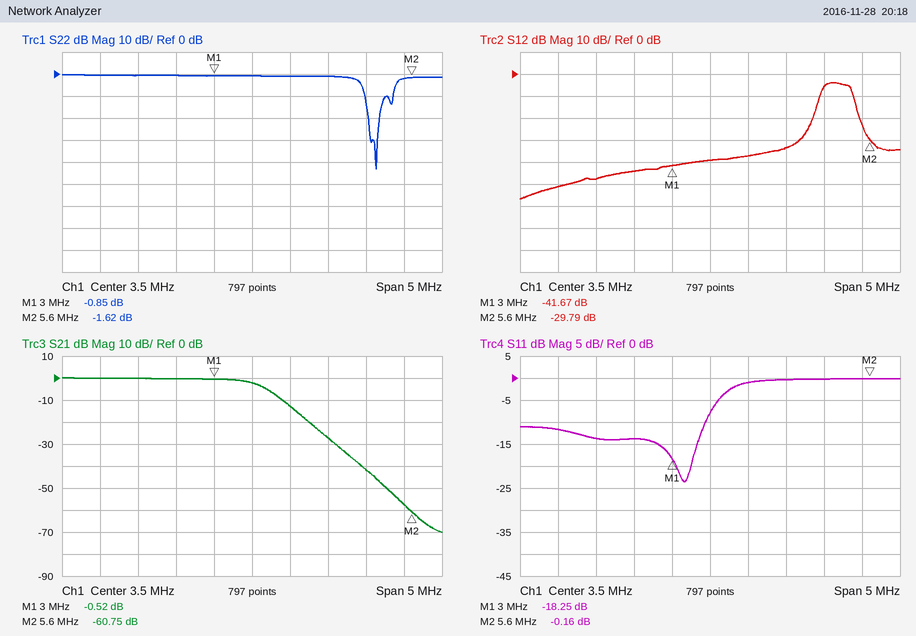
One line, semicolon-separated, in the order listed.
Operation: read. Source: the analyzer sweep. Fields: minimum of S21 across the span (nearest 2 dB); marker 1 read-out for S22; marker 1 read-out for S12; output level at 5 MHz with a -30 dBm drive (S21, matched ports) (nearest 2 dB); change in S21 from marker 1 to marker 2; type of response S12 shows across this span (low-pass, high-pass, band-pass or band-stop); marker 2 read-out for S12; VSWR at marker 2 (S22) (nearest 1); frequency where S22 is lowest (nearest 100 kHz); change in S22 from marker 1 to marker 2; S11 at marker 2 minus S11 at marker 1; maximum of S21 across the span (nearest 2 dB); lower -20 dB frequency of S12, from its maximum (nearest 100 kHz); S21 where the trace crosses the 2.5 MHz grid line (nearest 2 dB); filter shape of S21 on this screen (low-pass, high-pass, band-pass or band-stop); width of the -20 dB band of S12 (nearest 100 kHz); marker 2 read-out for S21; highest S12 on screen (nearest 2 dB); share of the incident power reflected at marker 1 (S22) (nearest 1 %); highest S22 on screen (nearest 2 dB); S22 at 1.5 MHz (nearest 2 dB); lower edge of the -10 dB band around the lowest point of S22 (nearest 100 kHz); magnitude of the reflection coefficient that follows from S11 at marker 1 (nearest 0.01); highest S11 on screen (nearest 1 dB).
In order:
-70 dB; -0.85 dB; -41.67 dB; -72 dBm; -60.23 dB; band-pass; -29.79 dB; 11; 5.1 MHz; -0.77 dB; 18.09 dB; 0 dB; 4.8 MHz; 0 dB; low-pass; 700 kHz; -60.75 dB; -4 dB; 82 %; 0 dB; 0 dB; 5.0 MHz; 0.12; 0 dB
